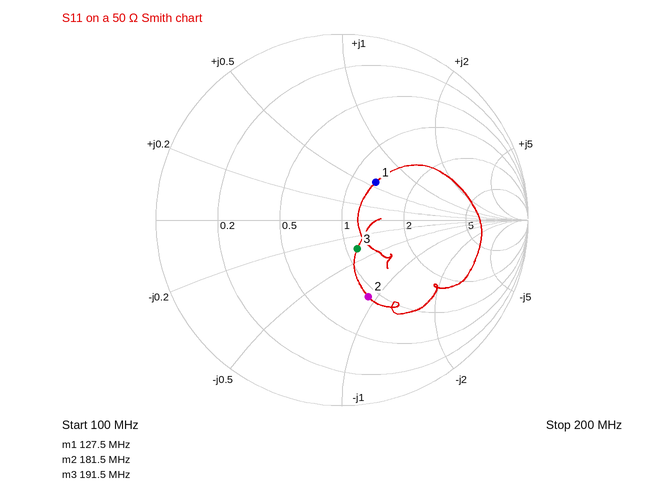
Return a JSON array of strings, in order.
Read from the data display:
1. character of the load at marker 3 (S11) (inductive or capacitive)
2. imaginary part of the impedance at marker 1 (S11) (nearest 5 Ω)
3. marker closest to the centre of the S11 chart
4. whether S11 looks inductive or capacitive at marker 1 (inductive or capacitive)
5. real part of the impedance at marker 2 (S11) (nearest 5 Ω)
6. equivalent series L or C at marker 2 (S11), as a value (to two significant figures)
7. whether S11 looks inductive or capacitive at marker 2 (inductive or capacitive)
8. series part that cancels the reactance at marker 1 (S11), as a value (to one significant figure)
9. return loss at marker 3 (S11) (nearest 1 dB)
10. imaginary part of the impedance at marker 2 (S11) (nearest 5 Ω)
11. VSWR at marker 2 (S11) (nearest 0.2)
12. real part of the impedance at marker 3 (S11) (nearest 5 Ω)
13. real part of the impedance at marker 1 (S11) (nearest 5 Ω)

["capacitive", "+30 Ω", "marker 3", "inductive", "45 Ω", "19 pF", "capacitive", "40 pF", "15 dB", "-45 Ω", "2.6", "55 Ω", "65 Ω"]
